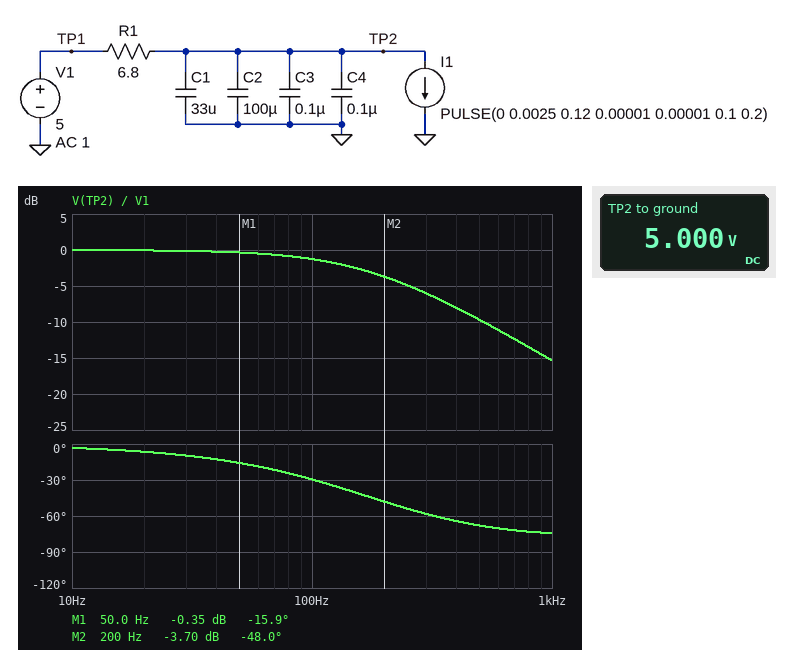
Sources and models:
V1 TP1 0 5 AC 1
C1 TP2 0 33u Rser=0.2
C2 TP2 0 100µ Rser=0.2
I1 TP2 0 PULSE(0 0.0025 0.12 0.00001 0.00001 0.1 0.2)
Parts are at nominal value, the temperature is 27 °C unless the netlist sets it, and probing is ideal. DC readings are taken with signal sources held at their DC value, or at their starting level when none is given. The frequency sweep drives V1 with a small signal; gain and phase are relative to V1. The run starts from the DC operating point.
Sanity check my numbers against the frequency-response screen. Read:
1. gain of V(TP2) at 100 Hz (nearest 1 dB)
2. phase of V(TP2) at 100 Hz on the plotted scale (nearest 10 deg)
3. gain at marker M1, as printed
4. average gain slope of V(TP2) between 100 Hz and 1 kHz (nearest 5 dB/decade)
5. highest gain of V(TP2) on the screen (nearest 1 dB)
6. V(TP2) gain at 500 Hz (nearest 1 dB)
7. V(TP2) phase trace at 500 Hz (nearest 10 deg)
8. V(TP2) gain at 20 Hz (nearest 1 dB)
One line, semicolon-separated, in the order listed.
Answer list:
-1 dB; -30 deg; -0.35 dB; -15 dB/decade; 0 dB; -10 dB; -70 deg; 0 dB
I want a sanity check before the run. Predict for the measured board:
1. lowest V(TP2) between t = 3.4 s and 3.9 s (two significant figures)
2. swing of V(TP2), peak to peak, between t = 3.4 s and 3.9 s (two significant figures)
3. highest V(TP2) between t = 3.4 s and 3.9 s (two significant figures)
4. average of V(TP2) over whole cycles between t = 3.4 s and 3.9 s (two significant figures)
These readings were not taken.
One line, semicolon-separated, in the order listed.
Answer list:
5.0 V; 17 mV; 5.0 V; 5.0 V
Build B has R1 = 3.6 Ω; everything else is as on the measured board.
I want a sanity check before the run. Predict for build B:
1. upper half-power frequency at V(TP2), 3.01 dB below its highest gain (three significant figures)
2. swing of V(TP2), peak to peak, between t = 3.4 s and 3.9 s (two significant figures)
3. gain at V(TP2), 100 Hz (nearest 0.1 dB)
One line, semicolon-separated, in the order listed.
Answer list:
321 Hz; 9.0 mV; -0.4 dB
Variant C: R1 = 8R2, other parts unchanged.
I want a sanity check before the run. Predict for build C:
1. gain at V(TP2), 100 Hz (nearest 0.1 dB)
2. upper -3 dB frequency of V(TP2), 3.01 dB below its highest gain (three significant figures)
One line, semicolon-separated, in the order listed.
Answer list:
-1.7 dB; 144 Hz
